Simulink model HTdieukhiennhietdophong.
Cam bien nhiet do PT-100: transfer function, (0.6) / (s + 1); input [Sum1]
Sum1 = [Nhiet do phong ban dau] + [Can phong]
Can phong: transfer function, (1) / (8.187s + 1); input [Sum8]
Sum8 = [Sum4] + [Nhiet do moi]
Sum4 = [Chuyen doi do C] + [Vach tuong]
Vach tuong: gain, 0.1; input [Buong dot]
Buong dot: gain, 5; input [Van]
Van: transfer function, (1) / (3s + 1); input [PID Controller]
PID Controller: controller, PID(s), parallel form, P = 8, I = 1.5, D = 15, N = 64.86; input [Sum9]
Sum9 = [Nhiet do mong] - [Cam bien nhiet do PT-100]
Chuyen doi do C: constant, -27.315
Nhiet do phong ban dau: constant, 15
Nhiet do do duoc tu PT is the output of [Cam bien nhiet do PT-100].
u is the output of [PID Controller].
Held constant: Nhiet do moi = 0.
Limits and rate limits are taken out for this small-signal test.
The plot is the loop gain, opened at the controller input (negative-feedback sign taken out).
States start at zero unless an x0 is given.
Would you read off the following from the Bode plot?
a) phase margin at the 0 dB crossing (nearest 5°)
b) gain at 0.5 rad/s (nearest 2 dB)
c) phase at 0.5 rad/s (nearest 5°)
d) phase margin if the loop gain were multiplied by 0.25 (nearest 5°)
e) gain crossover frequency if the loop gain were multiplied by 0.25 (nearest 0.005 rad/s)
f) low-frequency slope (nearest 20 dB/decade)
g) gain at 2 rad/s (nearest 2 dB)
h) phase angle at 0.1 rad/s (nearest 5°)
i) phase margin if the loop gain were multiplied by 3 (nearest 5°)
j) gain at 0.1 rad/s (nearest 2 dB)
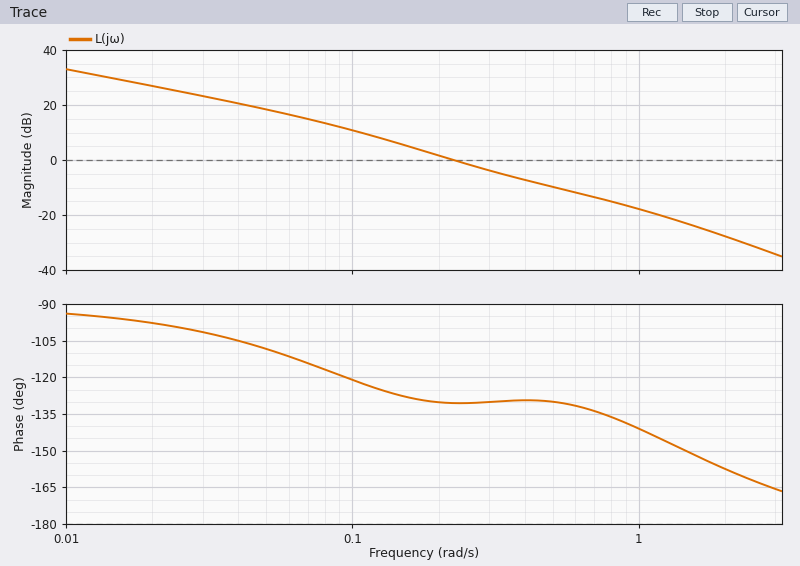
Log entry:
50°
-10 dB
-130°
60°
0.090 rad/s
-20 dB/decade
-28 dB
-120°
50°
10 dB
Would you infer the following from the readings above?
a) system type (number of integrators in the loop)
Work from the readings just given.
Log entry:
1
